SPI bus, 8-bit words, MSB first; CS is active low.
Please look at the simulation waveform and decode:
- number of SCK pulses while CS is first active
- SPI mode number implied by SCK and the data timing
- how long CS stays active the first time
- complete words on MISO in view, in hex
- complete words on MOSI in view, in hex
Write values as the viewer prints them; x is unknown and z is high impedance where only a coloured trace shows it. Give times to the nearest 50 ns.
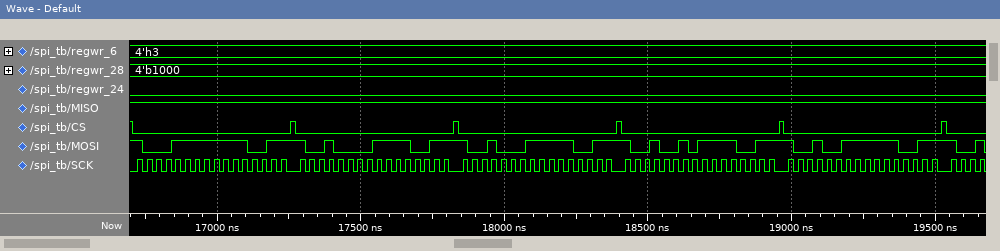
16
0
550 ns
FF, FF, FF, FF, FF, FF, FF, FF, FF, FF
8F, F3, 90, F3, 91, F3, 92, F3, 93, F3
